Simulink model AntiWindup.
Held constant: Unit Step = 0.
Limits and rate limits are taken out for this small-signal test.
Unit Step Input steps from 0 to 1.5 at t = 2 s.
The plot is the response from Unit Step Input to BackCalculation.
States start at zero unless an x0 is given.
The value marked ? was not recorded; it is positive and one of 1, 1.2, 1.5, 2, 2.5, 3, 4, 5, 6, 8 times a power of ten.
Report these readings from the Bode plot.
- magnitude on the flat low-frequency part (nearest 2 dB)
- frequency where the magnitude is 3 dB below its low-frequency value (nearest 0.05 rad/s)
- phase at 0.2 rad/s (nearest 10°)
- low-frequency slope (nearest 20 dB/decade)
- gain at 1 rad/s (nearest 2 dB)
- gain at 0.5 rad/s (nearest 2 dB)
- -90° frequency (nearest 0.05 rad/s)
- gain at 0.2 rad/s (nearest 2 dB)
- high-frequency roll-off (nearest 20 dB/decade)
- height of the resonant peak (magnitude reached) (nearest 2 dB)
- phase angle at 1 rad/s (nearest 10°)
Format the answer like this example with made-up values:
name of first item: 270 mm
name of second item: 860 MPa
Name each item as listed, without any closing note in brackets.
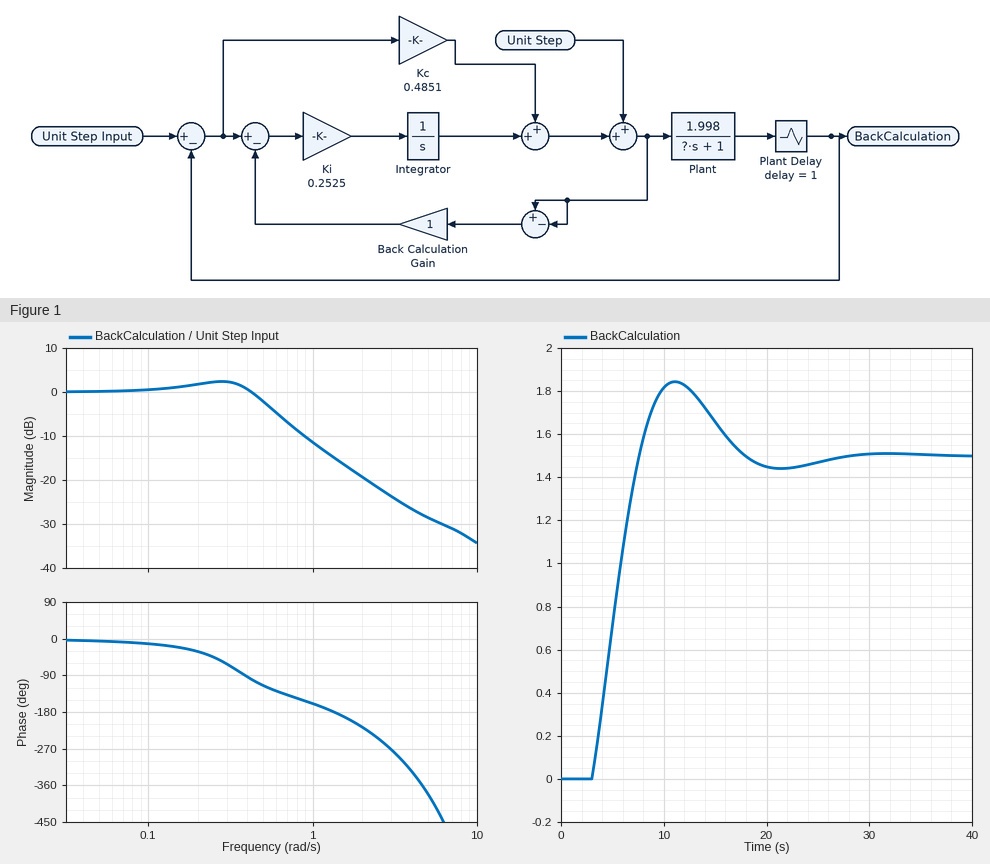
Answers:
magnitude on the flat low-frequency part: 0 dB
frequency where the magnitude is 3 dB below its low-frequency value: 0.55 rad/s
phase at 0.2 rad/s: -30°
low-frequency slope: 0 dB/decade
gain at 1 rad/s: -12 dB
gain at 0.5 rad/s: -2 dB
-90° frequency: 0.40 rad/s
gain at 0.2 rad/s: 2 dB
high-frequency roll-off: -20 dB/decade
height of the resonant peak (magnitude reached): 2 dB
phase angle at 1 rad/s: -160°
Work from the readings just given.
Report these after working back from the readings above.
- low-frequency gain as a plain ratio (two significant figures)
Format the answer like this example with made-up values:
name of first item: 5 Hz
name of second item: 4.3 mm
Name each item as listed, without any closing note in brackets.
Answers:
low-frequency gain as a plain ratio: 1.0
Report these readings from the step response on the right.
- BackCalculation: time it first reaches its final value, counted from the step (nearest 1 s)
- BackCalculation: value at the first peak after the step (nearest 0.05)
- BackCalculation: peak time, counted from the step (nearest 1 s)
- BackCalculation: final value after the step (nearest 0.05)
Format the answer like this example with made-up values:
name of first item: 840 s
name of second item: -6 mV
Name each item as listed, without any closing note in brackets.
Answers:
BackCalculation: time it first reaches its final value, counted from the step: 6 s
BackCalculation: value at the first peak after the step: 1.85
BackCalculation: peak time, counted from the step: 9 s
BackCalculation: final value after the step: 1.50
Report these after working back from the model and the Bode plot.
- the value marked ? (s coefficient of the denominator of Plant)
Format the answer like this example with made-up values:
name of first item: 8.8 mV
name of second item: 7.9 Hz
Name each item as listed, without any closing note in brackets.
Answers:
the value marked ?: 5
